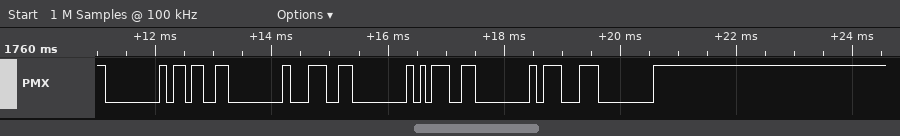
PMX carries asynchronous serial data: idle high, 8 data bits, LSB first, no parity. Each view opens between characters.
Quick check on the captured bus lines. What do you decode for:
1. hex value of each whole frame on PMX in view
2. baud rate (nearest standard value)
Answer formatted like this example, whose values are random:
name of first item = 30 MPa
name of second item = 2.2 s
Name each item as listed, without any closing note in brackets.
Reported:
hex value of each whole frame on PMX in view = 00, 9B, 00, 9C, 00, 9D, 00, C7, 00
baud rate = 9600 baud
